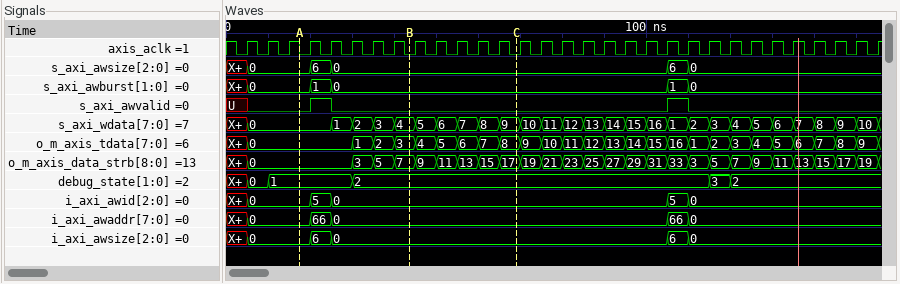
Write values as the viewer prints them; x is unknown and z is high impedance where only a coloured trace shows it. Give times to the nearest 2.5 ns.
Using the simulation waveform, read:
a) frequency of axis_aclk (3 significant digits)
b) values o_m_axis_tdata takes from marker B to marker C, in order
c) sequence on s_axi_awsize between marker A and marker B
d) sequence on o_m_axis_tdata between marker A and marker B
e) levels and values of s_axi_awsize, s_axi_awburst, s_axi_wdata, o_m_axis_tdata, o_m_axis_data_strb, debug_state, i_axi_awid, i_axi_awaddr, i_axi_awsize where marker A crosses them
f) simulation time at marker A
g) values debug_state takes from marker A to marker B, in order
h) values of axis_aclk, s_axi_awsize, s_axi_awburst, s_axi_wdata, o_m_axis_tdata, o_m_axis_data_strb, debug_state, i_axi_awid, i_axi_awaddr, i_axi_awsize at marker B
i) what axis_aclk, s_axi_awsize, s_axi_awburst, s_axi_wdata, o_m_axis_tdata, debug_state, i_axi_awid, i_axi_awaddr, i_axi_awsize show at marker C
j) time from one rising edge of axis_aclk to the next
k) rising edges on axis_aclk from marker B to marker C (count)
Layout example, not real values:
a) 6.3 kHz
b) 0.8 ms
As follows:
a) 200 MHz
b) 3, 4, 5, 6, 7, 8
c) 0, 6, 0
d) 0, 1, 2, 3
e) s_axi_awsize=0, s_axi_awburst=0, s_axi_wdata=0, o_m_axis_tdata=0, o_m_axis_data_strb=0, debug_state=1, i_axi_awid=0, i_axi_awaddr=0, i_axi_awsize=0
f) 17.5 ns
g) 1, 2
h) axis_aclk=0, s_axi_awsize=0, s_axi_awburst=0, s_axi_wdata=4, o_m_axis_tdata=3, o_m_axis_data_strb=7, debug_state=2, i_axi_awid=0, i_axi_awaddr=0, i_axi_awsize=0
i) axis_aclk=0, s_axi_awsize=0, s_axi_awburst=0, s_axi_wdata=9, o_m_axis_tdata=8, debug_state=2, i_axi_awid=0, i_axi_awaddr=0, i_axi_awsize=0
j) 5 ns
k) 5
